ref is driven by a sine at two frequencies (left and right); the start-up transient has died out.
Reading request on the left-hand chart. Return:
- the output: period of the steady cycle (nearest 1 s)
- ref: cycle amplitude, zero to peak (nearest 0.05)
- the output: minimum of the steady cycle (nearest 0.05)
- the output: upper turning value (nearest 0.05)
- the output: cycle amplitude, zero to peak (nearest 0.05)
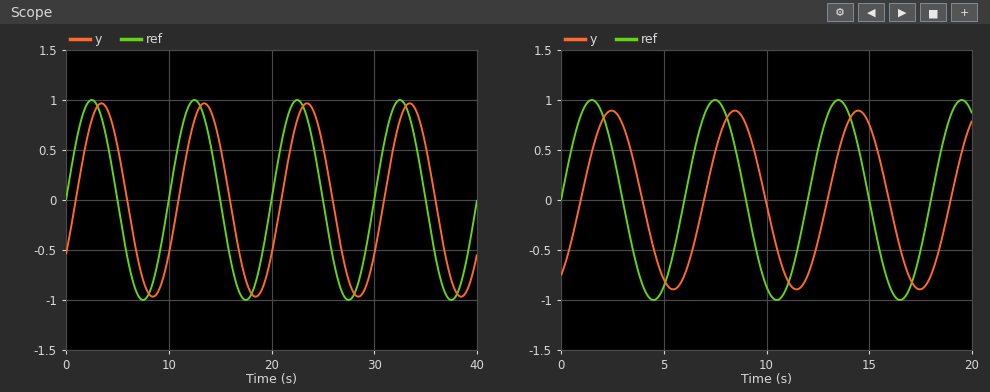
10 s
1.00
-0.95
0.95
0.95
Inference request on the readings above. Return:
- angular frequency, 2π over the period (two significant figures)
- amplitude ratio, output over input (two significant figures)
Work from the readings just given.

0.63 rad/s
0.95
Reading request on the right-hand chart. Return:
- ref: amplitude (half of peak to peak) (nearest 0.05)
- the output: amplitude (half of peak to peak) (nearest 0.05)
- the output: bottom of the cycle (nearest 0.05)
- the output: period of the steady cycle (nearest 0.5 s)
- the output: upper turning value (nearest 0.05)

1.00
0.90
-0.90
6.0 s
0.90
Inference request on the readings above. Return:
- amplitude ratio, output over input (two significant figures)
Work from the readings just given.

0.90
